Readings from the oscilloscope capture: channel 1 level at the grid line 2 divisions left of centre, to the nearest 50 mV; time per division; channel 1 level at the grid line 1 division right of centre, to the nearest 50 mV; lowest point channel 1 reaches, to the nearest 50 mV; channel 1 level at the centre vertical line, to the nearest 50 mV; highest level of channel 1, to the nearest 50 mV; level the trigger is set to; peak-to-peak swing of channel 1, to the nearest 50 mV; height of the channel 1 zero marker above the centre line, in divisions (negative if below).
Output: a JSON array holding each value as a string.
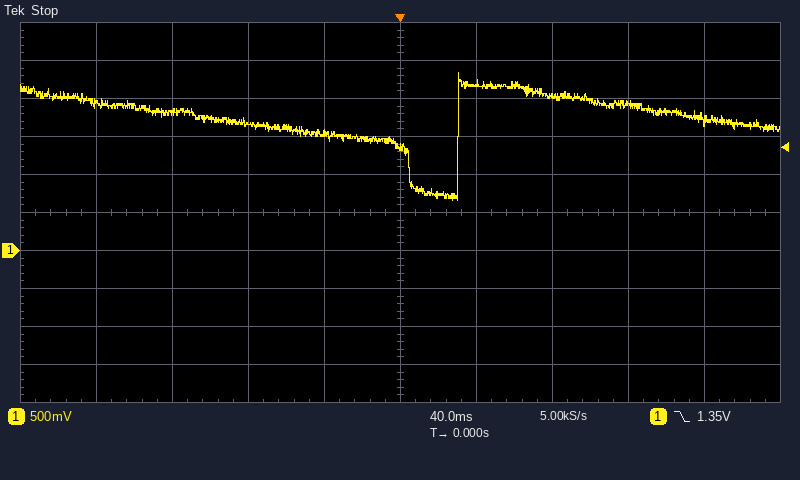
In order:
["1.65 V", "40 ms", "2.20 V", "650 mV", "1.35 V", "2.35 V", "1.35 V", "1.70 V", "-1.0 div"]
